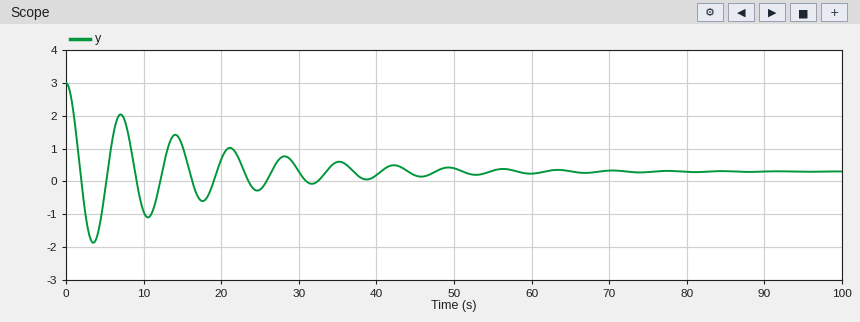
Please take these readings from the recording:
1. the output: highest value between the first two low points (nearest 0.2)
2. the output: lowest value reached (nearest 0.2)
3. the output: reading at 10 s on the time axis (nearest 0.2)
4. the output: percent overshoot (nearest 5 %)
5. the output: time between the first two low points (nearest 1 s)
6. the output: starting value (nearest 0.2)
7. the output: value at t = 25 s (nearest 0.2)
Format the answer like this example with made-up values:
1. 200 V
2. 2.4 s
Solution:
1. 2.0
2. -1.8
3. -1.0
4. 80 %
5. 7 s
6. 3.0
7. -0.2
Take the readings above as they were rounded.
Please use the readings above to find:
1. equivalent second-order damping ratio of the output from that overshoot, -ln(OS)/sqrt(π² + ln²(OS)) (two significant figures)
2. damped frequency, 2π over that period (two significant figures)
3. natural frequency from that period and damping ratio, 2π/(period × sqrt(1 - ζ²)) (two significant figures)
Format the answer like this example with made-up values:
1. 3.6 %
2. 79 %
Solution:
1. 0.071
2. 0.90 rad/s
3. 0.90 rad/s
